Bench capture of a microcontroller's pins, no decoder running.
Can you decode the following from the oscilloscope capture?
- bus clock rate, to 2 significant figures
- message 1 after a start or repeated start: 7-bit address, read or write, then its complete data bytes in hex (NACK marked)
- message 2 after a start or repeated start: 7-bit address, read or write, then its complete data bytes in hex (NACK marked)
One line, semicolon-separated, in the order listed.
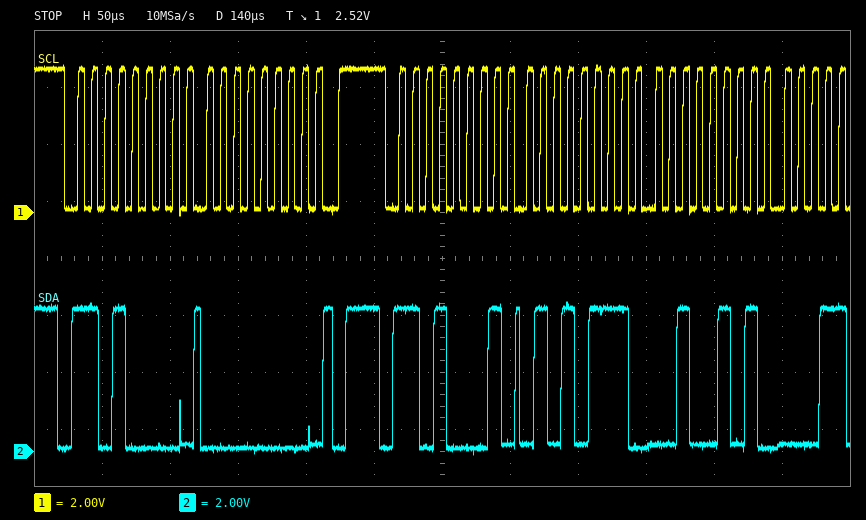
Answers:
100 kHz; 0x68 write: 00; 0x68 read: 57 25
